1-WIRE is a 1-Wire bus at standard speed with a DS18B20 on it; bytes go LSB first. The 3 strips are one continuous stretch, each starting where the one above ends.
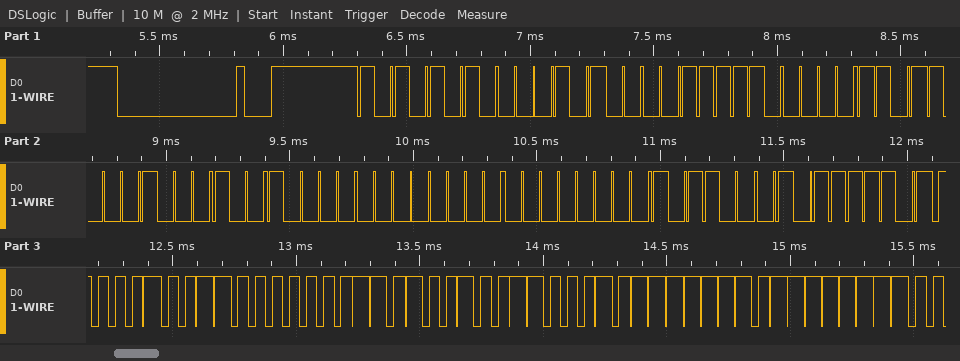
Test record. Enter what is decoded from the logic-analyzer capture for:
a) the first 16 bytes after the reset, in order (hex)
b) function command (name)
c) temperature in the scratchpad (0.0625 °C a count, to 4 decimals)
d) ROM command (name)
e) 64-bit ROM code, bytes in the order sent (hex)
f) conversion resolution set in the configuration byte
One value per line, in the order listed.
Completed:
55 28 7C B0 11 09 00 00 8D BE 90 01 4B 46 7F FF
Read Scratchpad
25.0000 °C
Match ROM
28 7C B0 11 09 00 00 8D
12 bits
